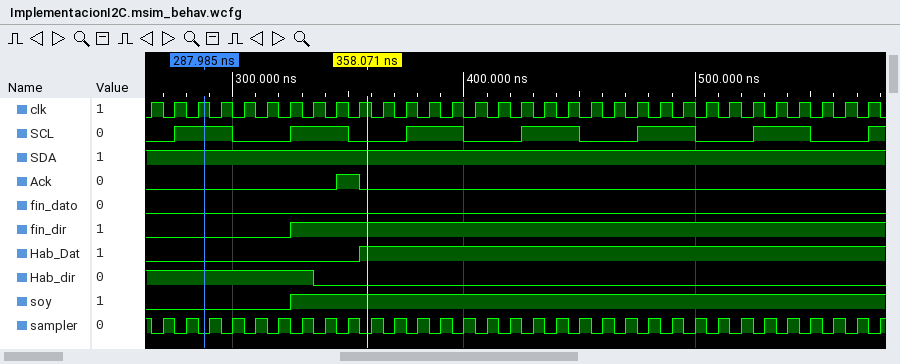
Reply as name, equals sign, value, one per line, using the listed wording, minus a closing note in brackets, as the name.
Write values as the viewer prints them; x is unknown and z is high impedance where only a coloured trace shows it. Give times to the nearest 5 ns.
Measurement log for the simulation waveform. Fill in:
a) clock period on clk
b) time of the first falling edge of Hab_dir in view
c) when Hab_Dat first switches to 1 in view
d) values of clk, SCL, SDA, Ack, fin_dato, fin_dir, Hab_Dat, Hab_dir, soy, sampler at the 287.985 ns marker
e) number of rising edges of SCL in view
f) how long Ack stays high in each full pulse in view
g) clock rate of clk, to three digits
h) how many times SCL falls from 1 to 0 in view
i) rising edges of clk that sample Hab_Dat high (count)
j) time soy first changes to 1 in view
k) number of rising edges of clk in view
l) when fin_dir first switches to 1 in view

clock period on clk = 10 ns
time of the first falling edge of Hab_dir in view = 335 ns
when Hab_Dat first switches to 1 in view = 355 ns
values of clk, SCL, SDA, Ack, fin_dato, fin_dir, Hab_Dat, Hab_dir, soy, sampler at the 287.985 ns marker = clk=1, SCL=1, SDA=1, Ack=0, fin_dato=0, fin_dir=0, Hab_Dat=0, Hab_dir=1, soy=0, sampler=0
number of rising edges of SCL in view = 7
how long Ack stays high in each full pulse in view = 10 ns
clock rate of clk, to three digits = 100 MHz
how many times SCL falls from 1 to 0 in view = 6
rising edges of clk that sample Hab_Dat high = 22
time soy first changes to 1 in view = 325 ns
number of rising edges of clk in view = 32
when fin_dir first switches to 1 in view = 325 ns
